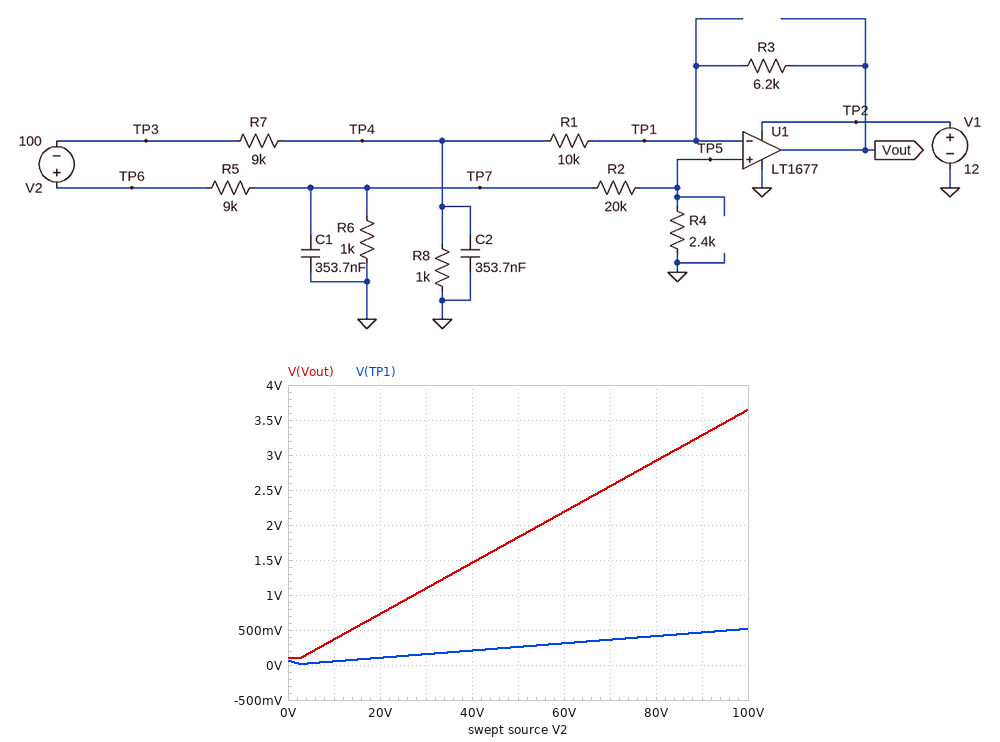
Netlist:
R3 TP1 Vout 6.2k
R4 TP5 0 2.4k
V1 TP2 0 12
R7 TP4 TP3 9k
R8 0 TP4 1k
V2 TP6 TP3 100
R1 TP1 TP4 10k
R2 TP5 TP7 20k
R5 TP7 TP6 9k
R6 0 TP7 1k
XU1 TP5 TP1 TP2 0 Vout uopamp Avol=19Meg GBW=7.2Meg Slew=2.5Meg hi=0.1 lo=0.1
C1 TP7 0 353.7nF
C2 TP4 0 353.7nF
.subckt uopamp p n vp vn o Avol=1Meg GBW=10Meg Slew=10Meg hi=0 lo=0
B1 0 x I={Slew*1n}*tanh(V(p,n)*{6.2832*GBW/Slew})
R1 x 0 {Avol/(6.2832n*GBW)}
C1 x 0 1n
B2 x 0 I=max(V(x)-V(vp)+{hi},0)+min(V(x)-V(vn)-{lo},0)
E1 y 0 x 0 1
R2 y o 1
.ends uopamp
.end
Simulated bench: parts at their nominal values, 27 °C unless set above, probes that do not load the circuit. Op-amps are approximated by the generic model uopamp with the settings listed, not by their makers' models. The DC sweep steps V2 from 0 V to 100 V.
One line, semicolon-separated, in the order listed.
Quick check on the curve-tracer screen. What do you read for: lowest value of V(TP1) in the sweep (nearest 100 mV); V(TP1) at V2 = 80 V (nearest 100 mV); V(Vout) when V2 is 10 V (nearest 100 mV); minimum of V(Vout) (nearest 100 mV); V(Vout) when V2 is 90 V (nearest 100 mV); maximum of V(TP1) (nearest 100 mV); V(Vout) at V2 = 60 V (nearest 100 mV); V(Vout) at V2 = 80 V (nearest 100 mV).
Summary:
0 V; 400 mV; 400 mV; 100 mV; 3.3 V; 500 mV; 2.2 V; 2.9 V
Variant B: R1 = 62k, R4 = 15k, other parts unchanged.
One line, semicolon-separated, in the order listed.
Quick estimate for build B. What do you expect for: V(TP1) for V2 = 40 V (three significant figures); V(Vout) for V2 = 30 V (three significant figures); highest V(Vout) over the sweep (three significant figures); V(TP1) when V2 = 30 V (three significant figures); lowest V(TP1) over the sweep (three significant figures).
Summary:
835 mV; 836 mV; 2.79 V; 627 mV; 75.2 mV
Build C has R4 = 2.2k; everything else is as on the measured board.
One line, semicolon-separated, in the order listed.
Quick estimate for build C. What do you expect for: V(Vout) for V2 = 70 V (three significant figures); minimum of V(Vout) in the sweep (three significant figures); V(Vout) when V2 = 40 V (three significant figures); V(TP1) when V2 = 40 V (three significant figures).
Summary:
2.51 V; 98.0 mV; 1.43 V; 191 mV
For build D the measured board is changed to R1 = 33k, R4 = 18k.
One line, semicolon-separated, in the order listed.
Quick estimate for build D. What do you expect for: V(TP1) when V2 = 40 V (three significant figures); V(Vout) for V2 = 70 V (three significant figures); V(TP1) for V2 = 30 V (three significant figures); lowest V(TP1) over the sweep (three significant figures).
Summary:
926 mV; 2.56 V; 695 mV; 63.7 mV
